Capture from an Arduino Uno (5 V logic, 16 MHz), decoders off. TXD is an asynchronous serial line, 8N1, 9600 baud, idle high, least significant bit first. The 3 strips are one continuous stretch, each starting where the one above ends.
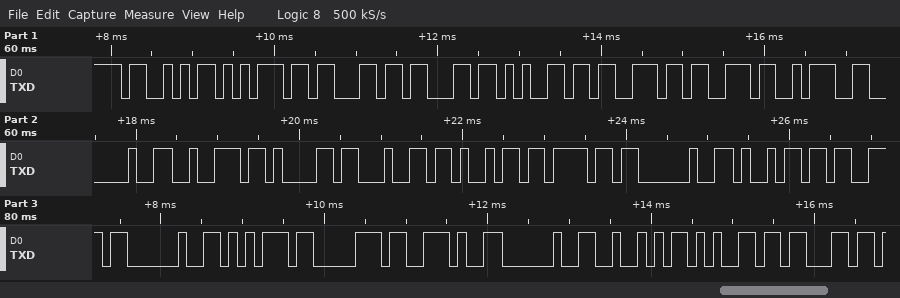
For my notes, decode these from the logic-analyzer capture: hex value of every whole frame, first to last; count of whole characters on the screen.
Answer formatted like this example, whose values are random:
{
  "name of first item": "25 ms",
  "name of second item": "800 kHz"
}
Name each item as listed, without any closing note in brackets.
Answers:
{
  "hex value of every whole frame, first to last": "53 75 63 63 65 73 73 3A 20 72 61 64 69 6F 20 69 73 20 75 70 2E 20 52 65 63",
  "count of whole characters on the screen": "25"
}
